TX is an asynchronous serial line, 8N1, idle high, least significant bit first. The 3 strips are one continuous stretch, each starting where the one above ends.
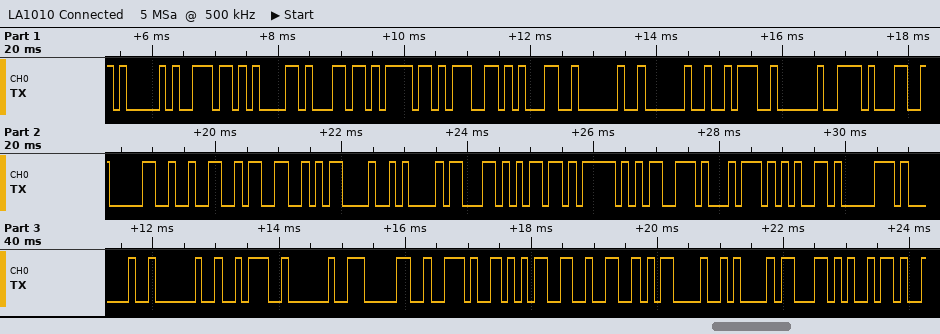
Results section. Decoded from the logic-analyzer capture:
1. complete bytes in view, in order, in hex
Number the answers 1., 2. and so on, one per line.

1. 41 6E 61 6C 6F 67 31 20 20 3A 20 31 30 32 33 0D 0A 63 6D 5F 73 74 65 70 20 20 3A 20 30 2E 35 32 0D 0A 63 69
